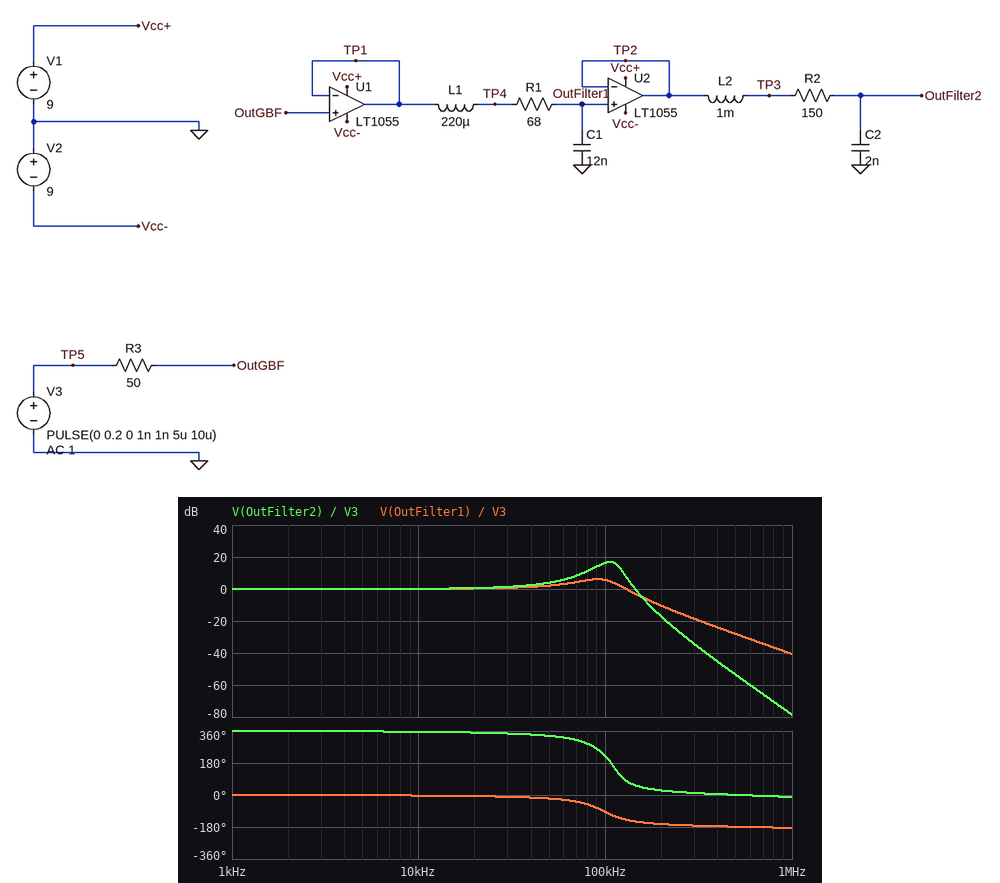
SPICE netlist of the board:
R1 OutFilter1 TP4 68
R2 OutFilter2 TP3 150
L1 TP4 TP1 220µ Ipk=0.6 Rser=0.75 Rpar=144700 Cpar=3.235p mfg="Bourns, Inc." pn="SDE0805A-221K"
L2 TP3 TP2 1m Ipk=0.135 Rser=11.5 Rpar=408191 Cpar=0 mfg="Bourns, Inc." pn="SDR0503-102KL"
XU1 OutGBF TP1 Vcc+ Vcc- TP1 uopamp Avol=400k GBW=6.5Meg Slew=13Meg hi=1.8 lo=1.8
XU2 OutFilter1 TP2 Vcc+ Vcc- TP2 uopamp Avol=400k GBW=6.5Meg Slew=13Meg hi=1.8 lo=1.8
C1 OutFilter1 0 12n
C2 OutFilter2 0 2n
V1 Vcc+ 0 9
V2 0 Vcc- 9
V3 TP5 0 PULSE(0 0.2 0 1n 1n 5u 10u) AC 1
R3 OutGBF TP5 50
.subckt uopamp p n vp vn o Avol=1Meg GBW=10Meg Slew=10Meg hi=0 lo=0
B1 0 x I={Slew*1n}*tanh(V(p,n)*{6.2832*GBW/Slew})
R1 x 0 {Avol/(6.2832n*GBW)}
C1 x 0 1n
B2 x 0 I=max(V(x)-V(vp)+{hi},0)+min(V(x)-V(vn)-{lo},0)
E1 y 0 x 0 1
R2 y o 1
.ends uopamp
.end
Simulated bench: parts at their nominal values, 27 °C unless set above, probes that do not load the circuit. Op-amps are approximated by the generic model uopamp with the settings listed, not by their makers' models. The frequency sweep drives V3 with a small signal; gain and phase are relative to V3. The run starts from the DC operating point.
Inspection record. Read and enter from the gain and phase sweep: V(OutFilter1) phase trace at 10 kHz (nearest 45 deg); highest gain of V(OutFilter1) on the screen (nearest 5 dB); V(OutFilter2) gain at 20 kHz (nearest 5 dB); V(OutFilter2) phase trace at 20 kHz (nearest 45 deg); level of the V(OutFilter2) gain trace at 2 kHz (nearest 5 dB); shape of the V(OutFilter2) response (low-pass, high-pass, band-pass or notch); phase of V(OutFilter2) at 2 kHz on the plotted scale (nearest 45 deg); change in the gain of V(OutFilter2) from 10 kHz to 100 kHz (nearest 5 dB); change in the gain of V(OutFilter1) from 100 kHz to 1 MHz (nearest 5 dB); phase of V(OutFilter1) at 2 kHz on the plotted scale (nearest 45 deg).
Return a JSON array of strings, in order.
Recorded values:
["0 deg", "5 dB", "0 dB", "360 deg", "0 dB", "low-pass", "360 deg", "15 dB", "-45 dB", "0 deg"]
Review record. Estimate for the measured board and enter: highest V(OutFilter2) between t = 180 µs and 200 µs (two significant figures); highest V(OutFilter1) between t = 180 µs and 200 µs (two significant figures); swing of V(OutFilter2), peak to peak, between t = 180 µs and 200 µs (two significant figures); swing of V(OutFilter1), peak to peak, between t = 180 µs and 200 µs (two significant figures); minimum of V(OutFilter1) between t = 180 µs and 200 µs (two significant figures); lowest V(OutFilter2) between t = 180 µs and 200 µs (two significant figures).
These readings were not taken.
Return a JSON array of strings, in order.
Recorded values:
["930 mV", "350 mV", "1.7 V", "500 mV", "-150 mV", "-730 mV"]
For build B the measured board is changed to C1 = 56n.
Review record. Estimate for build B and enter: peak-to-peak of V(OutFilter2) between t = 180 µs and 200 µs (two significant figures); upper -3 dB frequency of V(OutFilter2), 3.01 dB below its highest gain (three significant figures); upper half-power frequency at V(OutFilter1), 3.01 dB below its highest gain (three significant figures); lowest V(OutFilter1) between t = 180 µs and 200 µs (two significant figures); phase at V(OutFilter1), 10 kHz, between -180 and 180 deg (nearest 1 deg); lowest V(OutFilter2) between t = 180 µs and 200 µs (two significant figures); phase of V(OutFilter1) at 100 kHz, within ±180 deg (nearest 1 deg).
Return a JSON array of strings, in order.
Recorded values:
["190 mV", "60.7 kHz", "52.0 kHz", "72 mV", "-14 deg", "4.8 mV", "-149 deg"]
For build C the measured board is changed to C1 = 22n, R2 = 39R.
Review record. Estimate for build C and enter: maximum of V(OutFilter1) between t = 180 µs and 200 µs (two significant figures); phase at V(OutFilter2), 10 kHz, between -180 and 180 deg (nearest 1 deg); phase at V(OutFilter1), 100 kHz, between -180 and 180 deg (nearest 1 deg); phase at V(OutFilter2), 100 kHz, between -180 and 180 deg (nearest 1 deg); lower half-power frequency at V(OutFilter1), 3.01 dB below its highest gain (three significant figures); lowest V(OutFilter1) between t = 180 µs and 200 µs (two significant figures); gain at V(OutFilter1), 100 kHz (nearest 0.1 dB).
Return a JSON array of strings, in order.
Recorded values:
["200 mV", "-6 deg", "-135 deg", "-153 deg", "24.8 kHz", "2.1 mV", "-2.4 dB"]
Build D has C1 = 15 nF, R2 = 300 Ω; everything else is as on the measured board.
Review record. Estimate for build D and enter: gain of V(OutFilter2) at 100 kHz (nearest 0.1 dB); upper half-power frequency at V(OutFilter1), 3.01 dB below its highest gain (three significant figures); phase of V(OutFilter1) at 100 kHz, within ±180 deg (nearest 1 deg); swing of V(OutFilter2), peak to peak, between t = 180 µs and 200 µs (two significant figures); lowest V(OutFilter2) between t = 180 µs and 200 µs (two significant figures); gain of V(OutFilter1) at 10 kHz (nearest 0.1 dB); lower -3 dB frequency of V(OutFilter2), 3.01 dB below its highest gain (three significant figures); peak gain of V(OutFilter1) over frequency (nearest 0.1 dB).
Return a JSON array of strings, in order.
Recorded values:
["9.9 dB", "103 kHz", "-116 deg", "800 mV", "-300 mV", "0.1 dB", "67.0 kHz", "5.3 dB"]
